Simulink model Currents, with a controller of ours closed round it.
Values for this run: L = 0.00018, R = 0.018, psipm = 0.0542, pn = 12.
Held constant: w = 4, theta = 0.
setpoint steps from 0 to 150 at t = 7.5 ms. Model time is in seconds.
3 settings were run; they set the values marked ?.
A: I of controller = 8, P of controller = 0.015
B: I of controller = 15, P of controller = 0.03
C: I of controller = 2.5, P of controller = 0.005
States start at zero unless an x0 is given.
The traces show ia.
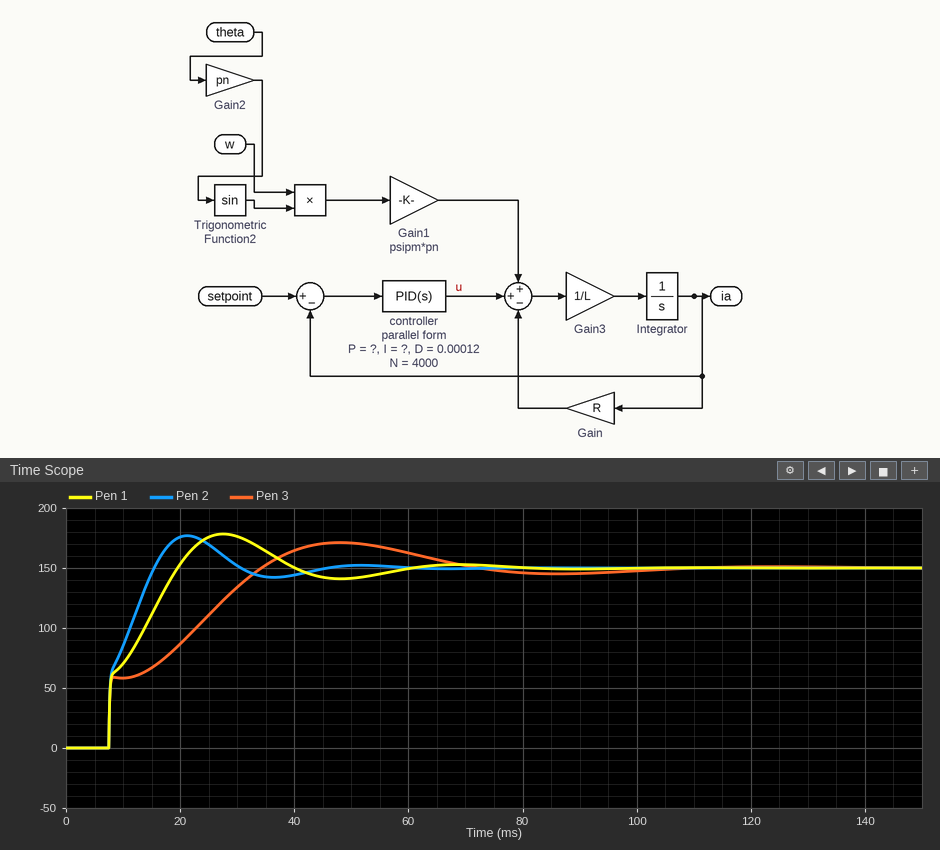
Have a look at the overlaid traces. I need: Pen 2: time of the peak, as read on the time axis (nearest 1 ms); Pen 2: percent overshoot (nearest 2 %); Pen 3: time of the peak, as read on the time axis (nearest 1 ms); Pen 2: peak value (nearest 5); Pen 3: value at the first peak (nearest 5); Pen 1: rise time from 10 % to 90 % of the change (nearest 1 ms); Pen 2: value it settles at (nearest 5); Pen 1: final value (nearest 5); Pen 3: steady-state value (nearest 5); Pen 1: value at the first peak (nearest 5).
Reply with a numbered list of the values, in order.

1. 21 ms
2. 18 %
3. 48 ms
4. 175
5. 170
6. 10 ms
7. 150
8. 150
9. 150
10. 180
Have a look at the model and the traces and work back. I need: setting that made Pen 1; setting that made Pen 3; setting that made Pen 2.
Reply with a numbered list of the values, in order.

1. A
2. C
3. B
